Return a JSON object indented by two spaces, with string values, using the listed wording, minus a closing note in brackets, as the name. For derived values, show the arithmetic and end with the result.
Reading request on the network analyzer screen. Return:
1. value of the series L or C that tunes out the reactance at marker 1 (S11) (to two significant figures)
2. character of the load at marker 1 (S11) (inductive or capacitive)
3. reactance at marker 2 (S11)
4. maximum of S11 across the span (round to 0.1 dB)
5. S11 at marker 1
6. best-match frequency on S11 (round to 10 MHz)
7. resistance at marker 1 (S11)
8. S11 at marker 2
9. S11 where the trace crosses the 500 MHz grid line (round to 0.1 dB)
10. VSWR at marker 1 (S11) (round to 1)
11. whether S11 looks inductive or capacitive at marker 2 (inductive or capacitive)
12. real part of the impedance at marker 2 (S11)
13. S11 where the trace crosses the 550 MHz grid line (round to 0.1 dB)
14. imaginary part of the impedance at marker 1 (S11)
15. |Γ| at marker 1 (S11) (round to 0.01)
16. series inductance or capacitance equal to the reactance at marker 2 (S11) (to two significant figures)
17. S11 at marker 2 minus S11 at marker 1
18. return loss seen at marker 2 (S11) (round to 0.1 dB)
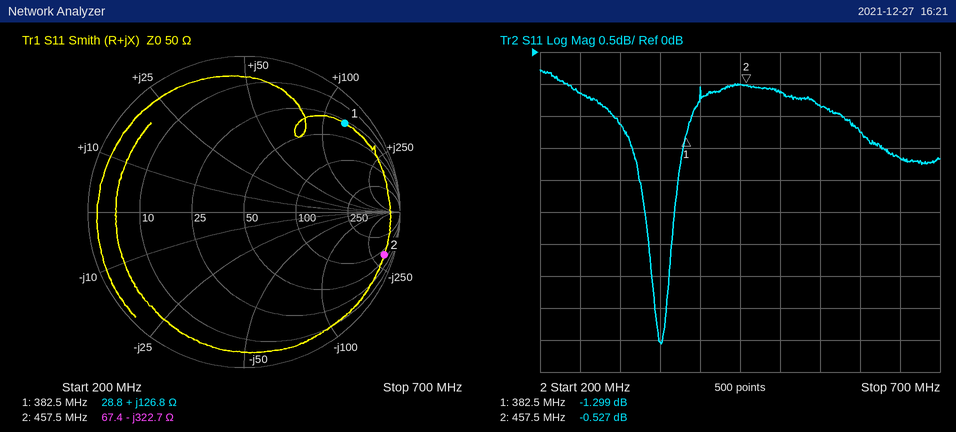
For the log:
{
  "value of the series L or C that tunes out the reactance at marker 1 (S11)": "C = 1/(2π × 382.5 MHz × 126.8 Ω) ≈ 3.3 pF",
  "character of the load at marker 1 (S11)": "inductive",
  "reactance at marker 2": "-322.7 Ω",
  "maximum of S11 across the span": "-0.3 dB",
  "S11 at marker 1": "-1.299 dB",
  "best-match frequency on S11": "350 MHz",
  "resistance at marker 1": "28.8 Ω",
  "S11 at marker 2": "-0.527 dB",
  "S11 where the trace crosses the 500 MHz grid line": "-0.6 dB",
  "VSWR at marker 1 (S11)": "(1 + 0.8611)/(1 − 0.8611) ≈ 13",
  "whether S11 looks inductive or capacitive at marker 2": "capacitive",
  "real part of the impedance at marker 2": "67.4 Ω",
  "S11 where the trace crosses the 550 MHz grid line": "-0.8 dB",
  "imaginary part of the impedance at marker 1": "+126.8 Ω",
  "|Γ| at marker 1 (S11)": "0.86",
  "series inductance or capacitance equal to the reactance at marker 2 (S11)": "C = 1/(2π × 457.5 MHz × 322.7 Ω) ≈ 1.1 pF",
  "S11 at marker 2 minus S11 at marker 1": "-0.527 − (-1.299) = 0.772 dB",
  "return loss seen at marker 2 (S11)": "0.5 dB"
}
